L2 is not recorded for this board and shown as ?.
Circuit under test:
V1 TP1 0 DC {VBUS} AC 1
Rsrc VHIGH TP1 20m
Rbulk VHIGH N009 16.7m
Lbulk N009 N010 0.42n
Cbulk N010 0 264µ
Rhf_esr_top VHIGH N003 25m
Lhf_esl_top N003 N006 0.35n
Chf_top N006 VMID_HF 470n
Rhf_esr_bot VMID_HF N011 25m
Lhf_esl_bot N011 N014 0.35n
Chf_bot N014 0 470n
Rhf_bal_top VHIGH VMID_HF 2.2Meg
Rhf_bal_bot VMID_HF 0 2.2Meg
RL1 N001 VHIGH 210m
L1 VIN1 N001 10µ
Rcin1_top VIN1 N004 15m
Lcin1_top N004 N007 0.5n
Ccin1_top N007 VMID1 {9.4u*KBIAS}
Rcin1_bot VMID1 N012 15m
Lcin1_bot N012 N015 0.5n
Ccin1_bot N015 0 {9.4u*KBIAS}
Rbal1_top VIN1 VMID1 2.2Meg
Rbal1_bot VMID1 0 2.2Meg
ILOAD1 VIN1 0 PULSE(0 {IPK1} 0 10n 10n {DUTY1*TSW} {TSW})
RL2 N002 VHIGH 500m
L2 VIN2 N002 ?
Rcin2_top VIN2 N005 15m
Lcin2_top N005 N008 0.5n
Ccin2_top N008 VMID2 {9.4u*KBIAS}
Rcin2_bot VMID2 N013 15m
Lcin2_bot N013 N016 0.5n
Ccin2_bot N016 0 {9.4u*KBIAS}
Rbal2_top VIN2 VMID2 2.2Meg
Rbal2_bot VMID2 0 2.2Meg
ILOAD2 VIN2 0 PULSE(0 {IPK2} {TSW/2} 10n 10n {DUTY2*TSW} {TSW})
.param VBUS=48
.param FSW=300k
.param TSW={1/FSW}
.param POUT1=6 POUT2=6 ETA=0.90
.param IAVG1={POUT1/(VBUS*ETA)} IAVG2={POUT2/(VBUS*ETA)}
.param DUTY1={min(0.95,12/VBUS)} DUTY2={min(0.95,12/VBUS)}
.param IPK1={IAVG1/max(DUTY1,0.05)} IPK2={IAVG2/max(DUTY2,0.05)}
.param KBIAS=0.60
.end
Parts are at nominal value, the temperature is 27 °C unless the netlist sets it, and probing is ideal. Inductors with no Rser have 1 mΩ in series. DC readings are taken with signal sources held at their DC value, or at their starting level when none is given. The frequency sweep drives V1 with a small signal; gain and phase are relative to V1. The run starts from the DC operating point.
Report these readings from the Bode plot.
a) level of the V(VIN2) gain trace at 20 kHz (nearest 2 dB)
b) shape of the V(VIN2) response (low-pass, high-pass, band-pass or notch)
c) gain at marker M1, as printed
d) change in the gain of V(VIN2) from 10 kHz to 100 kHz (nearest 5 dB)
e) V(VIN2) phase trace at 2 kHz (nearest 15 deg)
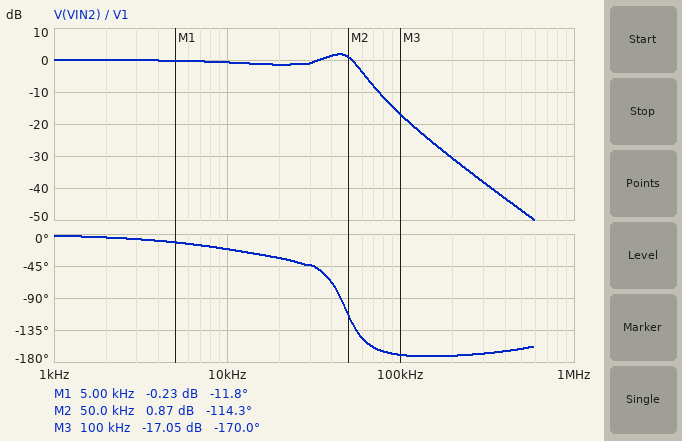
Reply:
-2 dB
low-pass
-0.23 dB
-15 dB
0 deg
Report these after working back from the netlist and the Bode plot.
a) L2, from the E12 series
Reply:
3.9 µH
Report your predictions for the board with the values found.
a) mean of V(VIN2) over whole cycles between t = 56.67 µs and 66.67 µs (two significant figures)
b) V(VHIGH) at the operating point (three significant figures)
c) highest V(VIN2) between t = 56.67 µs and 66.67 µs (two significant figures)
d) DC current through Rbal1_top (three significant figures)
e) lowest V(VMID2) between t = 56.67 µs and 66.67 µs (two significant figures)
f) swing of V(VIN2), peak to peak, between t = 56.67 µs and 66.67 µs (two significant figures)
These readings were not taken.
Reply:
48 V
48.0 V
48 V
10.9 µA
24 V
140 mV
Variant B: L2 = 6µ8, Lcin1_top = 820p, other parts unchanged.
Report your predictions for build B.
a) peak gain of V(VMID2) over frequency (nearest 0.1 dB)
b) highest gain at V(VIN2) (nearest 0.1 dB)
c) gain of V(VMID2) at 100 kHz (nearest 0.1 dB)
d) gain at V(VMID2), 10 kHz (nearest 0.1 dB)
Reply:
-1.3 dB
4.7 dB
-28.7 dB
-6.5 dB
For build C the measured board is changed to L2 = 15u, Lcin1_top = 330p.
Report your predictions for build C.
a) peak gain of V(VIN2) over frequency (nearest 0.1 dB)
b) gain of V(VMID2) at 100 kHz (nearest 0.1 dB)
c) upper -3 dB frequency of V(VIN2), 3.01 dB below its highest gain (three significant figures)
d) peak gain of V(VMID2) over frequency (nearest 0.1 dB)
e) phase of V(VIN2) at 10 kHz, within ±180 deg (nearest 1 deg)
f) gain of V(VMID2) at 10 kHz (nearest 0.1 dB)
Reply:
9.1 dB
-36.2 dB
26.7 kHz
3.1 dB
-22 deg
-5.6 dB
